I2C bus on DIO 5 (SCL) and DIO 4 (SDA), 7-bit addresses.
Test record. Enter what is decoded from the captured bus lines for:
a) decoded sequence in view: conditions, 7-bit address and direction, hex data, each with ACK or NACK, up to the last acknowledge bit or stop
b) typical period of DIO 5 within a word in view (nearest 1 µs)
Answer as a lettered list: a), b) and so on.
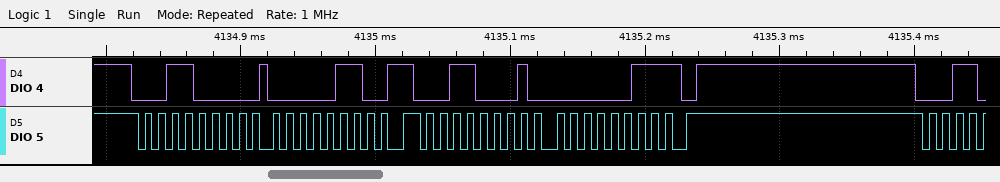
a) start, address 18 write ACK, 06 ACK, repeated start, address 18 read ACK, 03 NACK, stop
b) 10 µs
